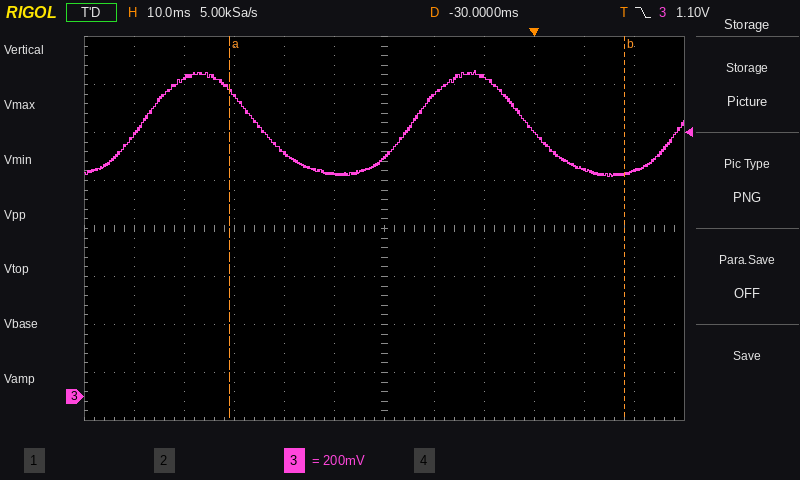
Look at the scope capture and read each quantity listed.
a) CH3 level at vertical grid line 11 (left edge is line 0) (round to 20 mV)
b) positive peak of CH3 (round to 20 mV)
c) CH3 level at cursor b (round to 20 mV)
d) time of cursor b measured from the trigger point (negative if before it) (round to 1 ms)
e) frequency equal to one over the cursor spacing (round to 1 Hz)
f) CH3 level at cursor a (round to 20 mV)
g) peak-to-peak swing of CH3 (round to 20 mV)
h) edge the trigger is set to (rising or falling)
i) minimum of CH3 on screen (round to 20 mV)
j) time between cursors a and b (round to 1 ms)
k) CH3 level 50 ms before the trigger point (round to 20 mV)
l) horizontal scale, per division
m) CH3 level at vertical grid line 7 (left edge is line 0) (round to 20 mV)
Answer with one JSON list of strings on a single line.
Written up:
["940 mV", "1.36 V", "920 mV", "+18 ms", "13 Hz", "1.28 V", "440 mV", "falling", "920 mV", "79 ms", "1.02 V", "10 ms", "1.26 V"]
